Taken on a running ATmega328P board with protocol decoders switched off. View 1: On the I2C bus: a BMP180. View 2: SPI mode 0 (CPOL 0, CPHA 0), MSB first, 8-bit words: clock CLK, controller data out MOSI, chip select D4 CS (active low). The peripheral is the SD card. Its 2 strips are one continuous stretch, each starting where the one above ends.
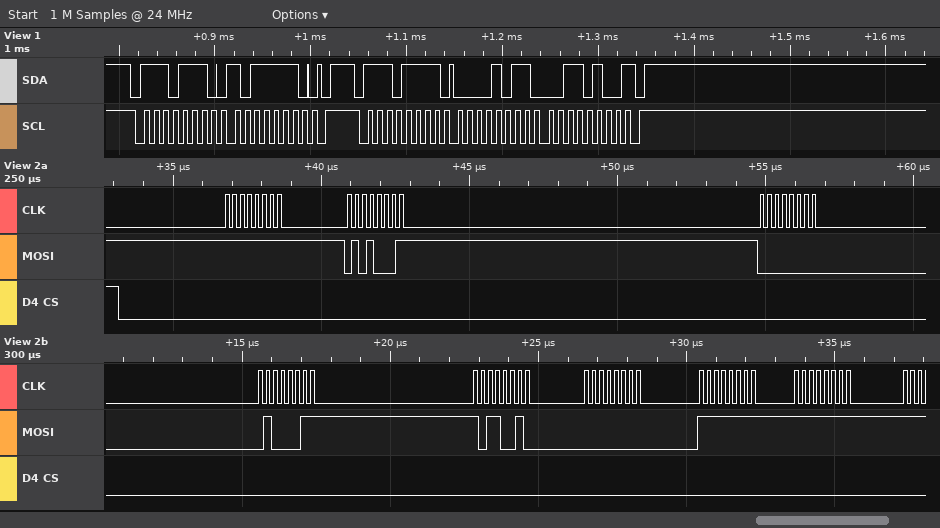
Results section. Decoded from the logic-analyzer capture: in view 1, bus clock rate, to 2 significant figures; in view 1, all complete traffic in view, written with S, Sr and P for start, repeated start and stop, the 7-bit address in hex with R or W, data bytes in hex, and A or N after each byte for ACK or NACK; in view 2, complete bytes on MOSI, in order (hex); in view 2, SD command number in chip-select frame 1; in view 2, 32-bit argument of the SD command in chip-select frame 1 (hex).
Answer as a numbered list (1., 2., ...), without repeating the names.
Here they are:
1. 100 kHz
2. S 77W A BE A P S 77R A 0B A 34 N P
3. FF 51 00 43 B2 00 FF FF
4. CMD17
5. 0x0043B200
